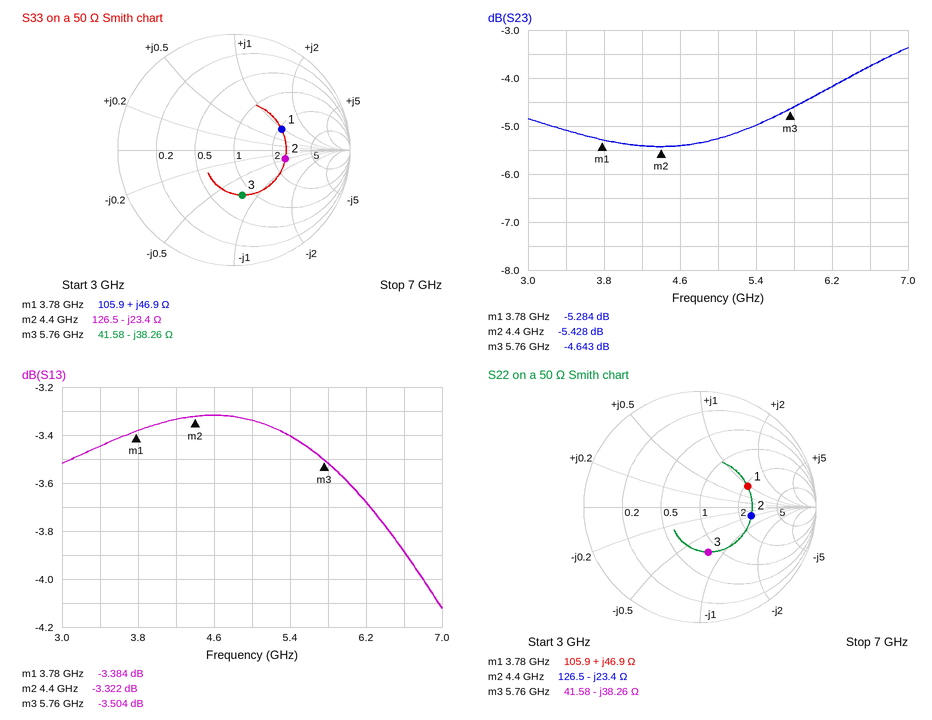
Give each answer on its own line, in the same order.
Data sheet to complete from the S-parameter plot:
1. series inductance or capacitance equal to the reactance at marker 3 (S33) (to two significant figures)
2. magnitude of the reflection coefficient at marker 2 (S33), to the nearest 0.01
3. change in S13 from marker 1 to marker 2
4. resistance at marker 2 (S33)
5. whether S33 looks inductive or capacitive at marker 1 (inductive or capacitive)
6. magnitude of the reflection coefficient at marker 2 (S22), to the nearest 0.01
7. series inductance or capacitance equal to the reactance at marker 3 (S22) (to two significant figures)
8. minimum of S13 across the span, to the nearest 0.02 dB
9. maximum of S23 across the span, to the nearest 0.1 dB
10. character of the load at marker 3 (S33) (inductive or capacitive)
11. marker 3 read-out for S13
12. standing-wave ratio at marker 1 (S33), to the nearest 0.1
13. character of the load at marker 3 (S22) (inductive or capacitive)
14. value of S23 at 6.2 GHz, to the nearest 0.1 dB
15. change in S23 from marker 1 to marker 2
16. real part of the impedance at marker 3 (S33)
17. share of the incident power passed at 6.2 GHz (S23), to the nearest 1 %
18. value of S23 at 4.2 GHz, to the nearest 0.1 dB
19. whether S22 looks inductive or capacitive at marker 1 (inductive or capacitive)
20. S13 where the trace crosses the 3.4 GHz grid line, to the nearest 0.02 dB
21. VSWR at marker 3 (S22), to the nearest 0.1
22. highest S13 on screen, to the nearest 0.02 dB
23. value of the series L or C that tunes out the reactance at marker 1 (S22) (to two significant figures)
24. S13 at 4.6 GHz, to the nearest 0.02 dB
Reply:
720 fF
0.45
0.062 dB
126.5 Ω
inductive
0.45
720 fF
-4.12 dB
-3.4 dB
capacitive
-3.504 dB
2.6
capacitive
-4.2 dB
-0.144 dB
41.58 Ω
38 %
-5.4 dB
inductive
-3.44 dB
2.3
-3.32 dB
900 fF
-3.32 dB
